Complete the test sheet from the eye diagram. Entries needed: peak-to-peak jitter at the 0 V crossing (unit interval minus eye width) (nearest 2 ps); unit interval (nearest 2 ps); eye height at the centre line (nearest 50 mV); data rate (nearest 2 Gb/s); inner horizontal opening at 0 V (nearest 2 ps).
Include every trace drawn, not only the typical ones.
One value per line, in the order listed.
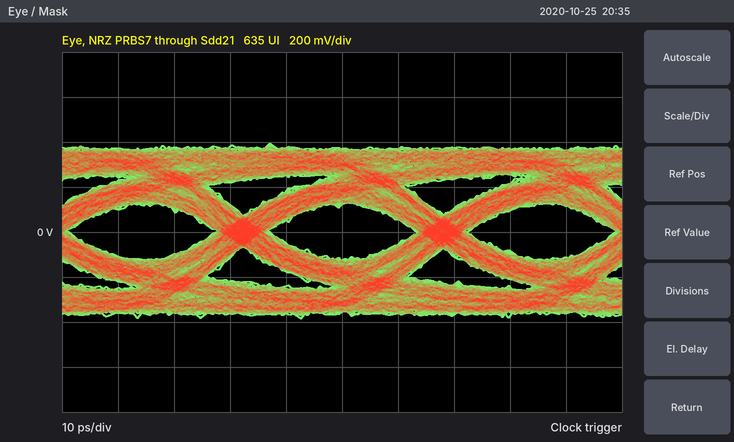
10 ps
36 ps
250 mV
28 Gb/s
26 ps
